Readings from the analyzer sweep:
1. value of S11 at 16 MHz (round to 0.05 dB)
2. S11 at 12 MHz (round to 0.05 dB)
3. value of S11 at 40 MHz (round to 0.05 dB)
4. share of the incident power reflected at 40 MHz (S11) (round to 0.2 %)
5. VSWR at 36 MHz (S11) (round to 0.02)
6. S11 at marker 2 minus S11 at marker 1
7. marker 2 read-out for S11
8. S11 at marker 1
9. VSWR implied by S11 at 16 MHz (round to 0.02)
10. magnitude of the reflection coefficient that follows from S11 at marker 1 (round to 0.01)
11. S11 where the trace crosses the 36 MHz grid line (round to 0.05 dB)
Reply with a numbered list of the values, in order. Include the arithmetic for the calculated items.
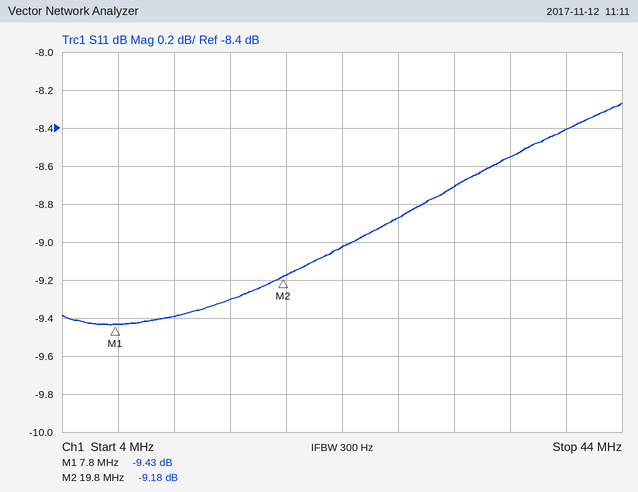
1. -9.30 dB
2. -9.40 dB
3. -8.40 dB
4. 10^(-8.4/10) ≈ 14.5 %, so 14.4 % to the nearest 0.2 %
5. |Γ| = 10^(-8.55/20) = 0.3737; VSWR = (1 + 0.3737)/(1 − 0.3737) ≈ 2.19, so 2.20 to the nearest 0.02
6. -9.18 − (-9.43) = 0.25 dB
7. -9.18 dB
8. -9.43 dB
9. |Γ| = 10^(-9.3/20) = 0.3428; VSWR = (1 + 0.3428)/(1 − 0.3428) ≈ 2.04
10. 10^(-9.43/20) ≈ 0.34
11. -8.55 dB
